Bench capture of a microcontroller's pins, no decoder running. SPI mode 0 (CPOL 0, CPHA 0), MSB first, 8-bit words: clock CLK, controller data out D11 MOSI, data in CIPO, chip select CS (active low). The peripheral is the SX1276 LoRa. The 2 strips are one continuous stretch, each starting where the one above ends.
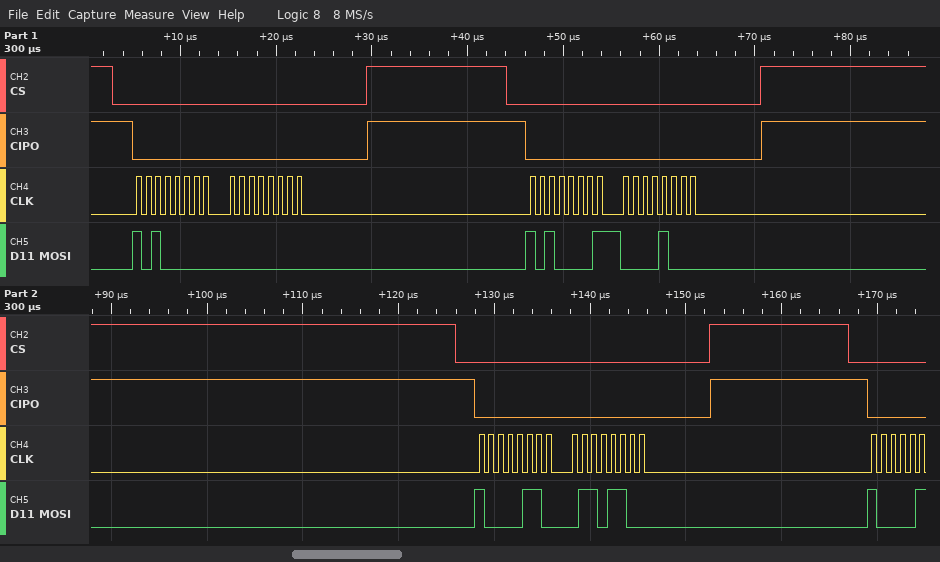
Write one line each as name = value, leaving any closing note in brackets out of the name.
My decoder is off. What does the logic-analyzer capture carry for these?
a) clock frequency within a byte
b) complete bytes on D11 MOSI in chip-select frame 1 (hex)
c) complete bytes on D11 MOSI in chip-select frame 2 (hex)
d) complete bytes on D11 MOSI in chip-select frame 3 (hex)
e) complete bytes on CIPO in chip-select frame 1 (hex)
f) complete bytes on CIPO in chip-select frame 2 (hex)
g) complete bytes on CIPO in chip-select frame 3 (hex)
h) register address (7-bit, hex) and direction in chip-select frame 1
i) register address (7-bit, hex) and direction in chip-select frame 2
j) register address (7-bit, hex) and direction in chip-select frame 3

clock frequency within a byte = 1 MHz
complete bytes on D11 MOSI in chip-select frame 1 = 0xA0 0x00
complete bytes on D11 MOSI in chip-select frame 2 = 0xA1 0x08
complete bytes on D11 MOSI in chip-select frame 3 = 0x86 0x6C
complete bytes on CIPO in chip-select frame 1 = 0x00 0x00
complete bytes on CIPO in chip-select frame 2 = 0x00 0x00
complete bytes on CIPO in chip-select frame 3 = 0x00 0x00
register address (7-bit, hex) and direction in chip-select frame 1 = 0x20 write
register address (7-bit, hex) and direction in chip-select frame 2 = 0x21 write
register address (7-bit, hex) and direction in chip-select frame 3 = 0x06 write
